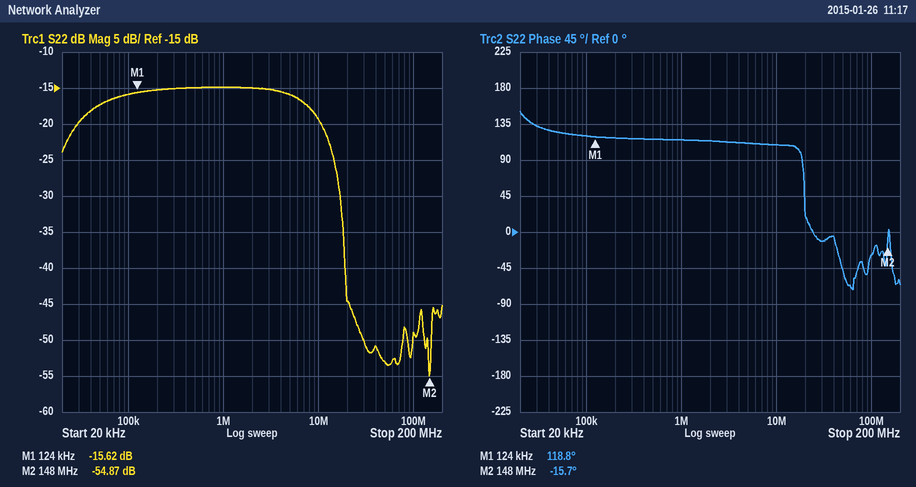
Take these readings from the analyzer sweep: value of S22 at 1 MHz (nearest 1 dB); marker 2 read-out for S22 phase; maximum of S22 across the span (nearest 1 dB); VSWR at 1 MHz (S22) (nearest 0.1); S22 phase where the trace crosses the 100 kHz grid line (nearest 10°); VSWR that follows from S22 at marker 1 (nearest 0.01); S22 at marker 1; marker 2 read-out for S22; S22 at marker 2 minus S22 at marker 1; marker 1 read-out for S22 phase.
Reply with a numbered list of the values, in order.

1. -15 dB
2. -15.7°
3. -15 dB
4. 1.4
5. 120°
6. 1.40
7. -15.62 dB
8. -54.87 dB
9. -39.25 dB
10. 118.8°
